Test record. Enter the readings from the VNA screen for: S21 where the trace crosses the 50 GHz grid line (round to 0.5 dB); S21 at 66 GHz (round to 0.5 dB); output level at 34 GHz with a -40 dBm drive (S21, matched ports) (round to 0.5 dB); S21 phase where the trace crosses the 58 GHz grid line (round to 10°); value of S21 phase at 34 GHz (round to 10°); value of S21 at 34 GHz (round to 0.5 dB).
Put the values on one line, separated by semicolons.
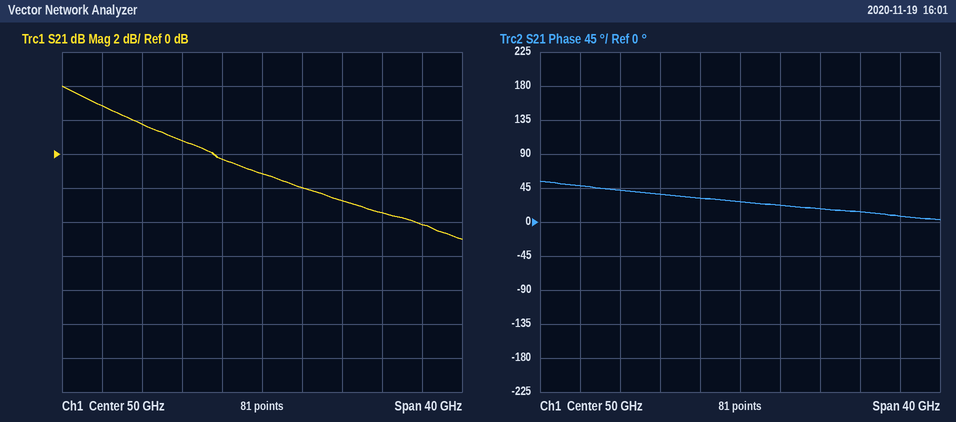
-1.0 dB; -4.0 dB; -37.0 dBm; 20°; 50°; 3.0 dB
